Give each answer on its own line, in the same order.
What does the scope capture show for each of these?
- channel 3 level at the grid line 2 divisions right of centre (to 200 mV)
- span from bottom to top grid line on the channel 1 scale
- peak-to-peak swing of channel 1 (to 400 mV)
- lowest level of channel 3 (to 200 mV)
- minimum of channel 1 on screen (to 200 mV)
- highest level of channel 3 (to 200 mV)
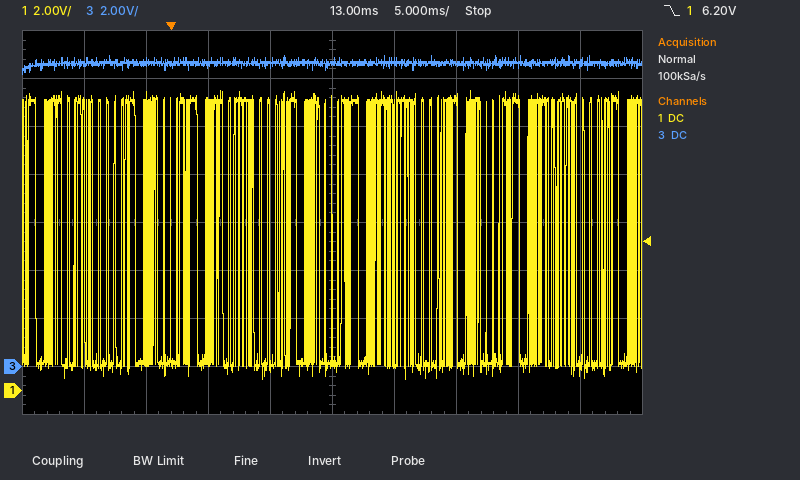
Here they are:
12.6 V
16 V
12.0 V
12.2 V
400 mV
13.0 V
